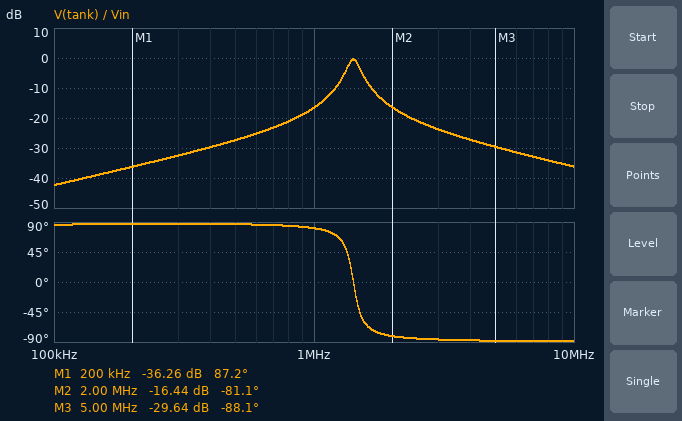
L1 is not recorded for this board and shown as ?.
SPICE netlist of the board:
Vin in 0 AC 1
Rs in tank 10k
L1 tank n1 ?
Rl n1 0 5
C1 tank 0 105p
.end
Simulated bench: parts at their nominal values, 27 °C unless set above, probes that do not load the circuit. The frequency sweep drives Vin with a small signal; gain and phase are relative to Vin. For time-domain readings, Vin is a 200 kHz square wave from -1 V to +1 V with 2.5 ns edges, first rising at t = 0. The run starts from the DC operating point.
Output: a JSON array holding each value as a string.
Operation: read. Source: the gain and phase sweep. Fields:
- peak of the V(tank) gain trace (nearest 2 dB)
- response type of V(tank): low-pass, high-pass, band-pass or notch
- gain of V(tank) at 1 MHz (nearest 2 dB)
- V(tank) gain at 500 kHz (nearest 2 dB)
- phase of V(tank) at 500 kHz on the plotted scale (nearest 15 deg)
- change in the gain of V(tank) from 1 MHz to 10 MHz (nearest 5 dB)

["0 dB", "band-pass", "-16 dB", "-28 dB", "90 deg", "-20 dB"]
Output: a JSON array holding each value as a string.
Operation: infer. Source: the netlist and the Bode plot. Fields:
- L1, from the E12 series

["120 µH"]
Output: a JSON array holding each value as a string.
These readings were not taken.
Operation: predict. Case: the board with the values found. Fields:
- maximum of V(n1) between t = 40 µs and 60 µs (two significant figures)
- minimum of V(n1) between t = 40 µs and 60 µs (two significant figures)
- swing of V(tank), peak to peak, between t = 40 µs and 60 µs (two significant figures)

["1.7 mV", "-1.7 mV", "550 mV"]
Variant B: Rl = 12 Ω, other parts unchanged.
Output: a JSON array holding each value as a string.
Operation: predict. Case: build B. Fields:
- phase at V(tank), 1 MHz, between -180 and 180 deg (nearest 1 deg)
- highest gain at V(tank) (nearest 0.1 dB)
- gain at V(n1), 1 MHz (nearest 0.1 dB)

["80 deg", "-0.9 dB", "-52.6 dB"]
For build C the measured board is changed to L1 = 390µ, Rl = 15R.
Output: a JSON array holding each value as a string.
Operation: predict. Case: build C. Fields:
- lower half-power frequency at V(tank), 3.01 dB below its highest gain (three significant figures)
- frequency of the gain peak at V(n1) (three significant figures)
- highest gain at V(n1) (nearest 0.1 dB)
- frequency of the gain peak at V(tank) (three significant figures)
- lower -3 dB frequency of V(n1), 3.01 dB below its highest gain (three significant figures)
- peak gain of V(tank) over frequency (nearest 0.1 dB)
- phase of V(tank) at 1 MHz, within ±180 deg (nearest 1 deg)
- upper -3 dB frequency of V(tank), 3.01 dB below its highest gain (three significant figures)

["712 kHz", "779 kHz", "-42.5 dB", "787 kHz", "695 kHz", "-0.3 dB", "-68 deg", "870 kHz"]
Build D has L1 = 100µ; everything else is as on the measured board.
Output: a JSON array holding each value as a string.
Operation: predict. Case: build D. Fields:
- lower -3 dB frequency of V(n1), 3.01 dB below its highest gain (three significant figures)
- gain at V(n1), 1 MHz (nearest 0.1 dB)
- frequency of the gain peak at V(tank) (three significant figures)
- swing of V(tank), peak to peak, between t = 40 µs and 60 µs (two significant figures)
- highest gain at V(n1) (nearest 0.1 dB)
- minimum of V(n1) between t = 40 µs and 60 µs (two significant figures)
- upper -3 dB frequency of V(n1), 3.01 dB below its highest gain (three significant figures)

["1.47 MHz", "-61.4 dB", "1.55 MHz", "300 mV", "-46.2 dB", "-1.2 mV", "1.63 MHz"]
